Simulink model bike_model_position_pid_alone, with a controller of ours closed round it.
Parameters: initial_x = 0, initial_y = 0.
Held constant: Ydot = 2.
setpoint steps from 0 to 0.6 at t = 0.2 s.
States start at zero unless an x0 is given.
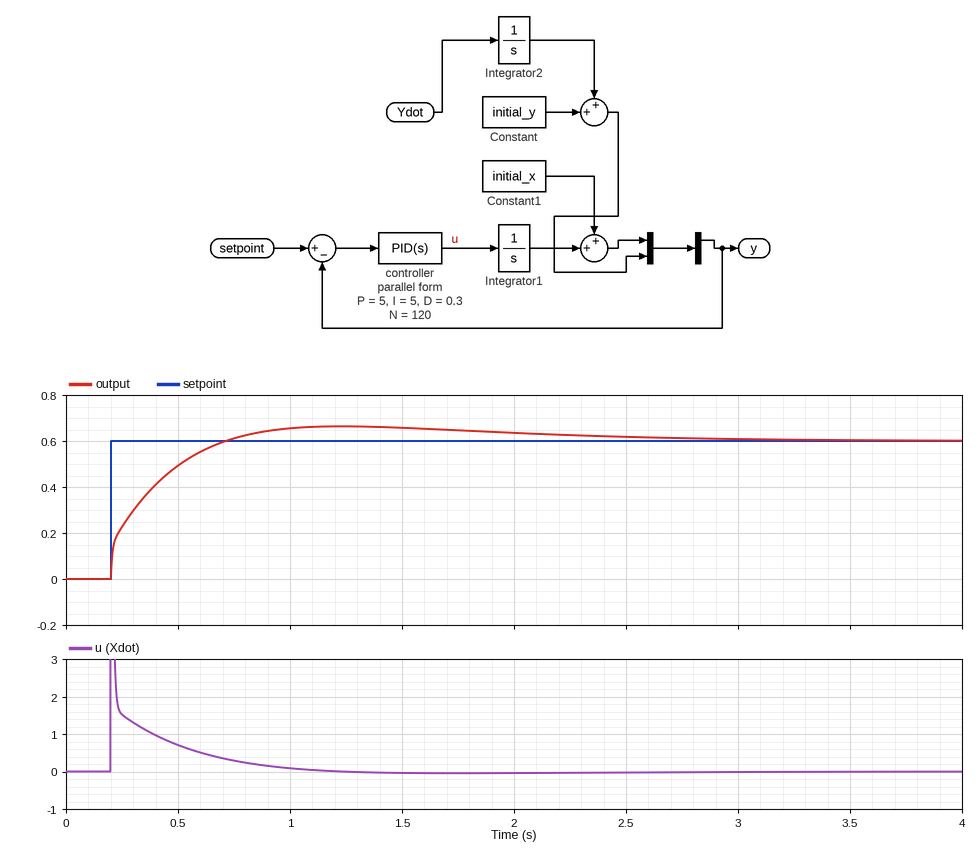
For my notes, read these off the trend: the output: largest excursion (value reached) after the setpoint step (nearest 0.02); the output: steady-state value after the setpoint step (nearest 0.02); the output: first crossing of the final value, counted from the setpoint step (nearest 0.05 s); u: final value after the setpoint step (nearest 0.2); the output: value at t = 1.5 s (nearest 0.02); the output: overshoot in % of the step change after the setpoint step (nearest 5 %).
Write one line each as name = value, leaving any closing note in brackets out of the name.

the output: largest excursion (value reached) after the setpoint step = 0.66
the output: steady-state value after the setpoint step = 0.60
the output: first crossing of the final value, counted from the setpoint step = 0.50 s
u: final value after the setpoint step = 0.0
the output: value at t = 1.5 s = 0.66
the output: overshoot in % of the step change after the setpoint step = 10 %
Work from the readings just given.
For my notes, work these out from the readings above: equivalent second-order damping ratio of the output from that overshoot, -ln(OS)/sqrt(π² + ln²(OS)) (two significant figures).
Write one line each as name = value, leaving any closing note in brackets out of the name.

equivalent second-order damping ratio of the output from that overshoot, -ln(OS)/sqrt(π² + ln²(OS)) = 0.59
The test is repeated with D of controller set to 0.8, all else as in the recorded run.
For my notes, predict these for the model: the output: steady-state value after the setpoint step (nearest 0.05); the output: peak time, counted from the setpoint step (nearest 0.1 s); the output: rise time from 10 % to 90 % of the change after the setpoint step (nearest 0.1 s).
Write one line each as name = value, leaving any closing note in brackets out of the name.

the output: steady-state value after the setpoint step = 0.60
the output: peak time, counted from the setpoint step = 1.3 s
the output: rise time from 10 % to 90 % of the change after the setpoint step = 0.4 s
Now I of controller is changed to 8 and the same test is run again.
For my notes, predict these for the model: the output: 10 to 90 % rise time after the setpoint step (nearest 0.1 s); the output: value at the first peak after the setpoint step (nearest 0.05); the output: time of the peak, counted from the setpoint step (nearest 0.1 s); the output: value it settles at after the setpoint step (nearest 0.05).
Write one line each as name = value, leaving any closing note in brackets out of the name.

the output: 10 to 90 % rise time after the setpoint step = 0.3 s
the output: value at the first peak after the setpoint step = 0.70
the output: time of the peak, counted from the setpoint step = 0.9 s
the output: value it settles at after the setpoint step = 0.60
